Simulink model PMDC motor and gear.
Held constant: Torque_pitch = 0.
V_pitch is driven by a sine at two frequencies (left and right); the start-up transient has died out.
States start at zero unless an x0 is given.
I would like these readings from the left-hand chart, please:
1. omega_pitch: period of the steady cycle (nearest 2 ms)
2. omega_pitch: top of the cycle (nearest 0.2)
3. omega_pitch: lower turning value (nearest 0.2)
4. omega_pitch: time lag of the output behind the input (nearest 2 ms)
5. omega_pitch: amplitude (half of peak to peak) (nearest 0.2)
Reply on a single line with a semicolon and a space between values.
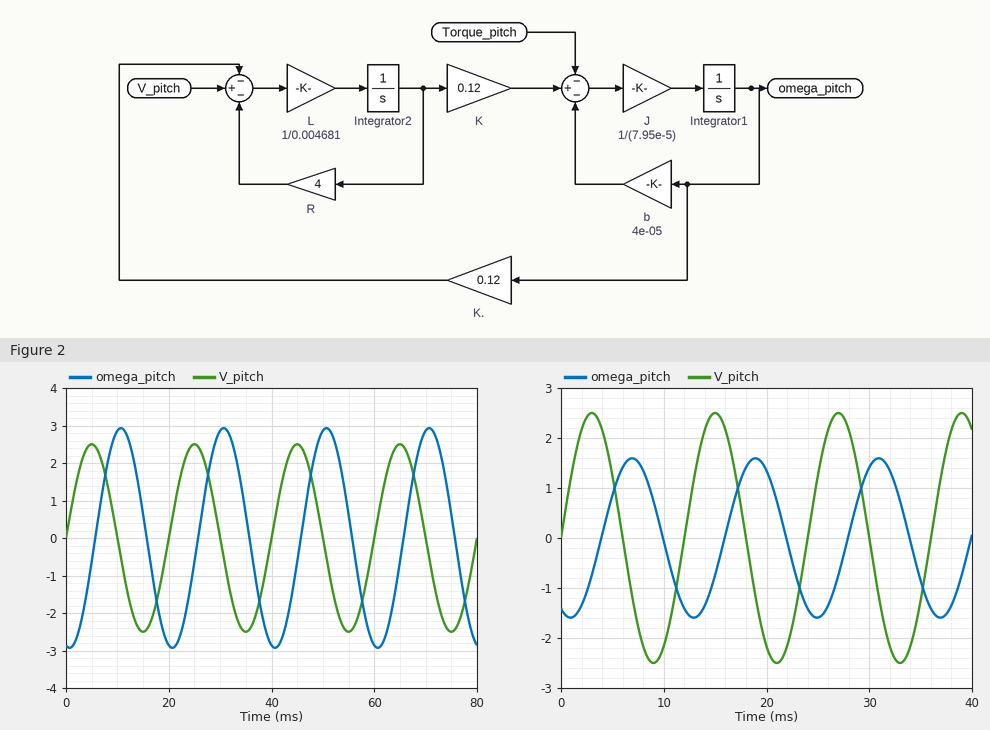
20 ms; 3.0; -3.0; 6 ms; 3.0
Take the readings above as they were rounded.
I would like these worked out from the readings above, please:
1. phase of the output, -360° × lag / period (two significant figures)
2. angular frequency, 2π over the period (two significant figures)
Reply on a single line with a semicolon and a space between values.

-110°; 0.31 rad/ms
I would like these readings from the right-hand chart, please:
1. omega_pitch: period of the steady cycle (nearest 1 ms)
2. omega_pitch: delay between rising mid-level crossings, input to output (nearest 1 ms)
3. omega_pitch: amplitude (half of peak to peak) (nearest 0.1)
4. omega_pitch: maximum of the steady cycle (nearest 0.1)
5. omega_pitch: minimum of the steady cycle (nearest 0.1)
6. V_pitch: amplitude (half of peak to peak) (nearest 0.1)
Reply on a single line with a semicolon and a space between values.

12 ms; 4 ms; 1.6; 1.6; -1.6; 2.5
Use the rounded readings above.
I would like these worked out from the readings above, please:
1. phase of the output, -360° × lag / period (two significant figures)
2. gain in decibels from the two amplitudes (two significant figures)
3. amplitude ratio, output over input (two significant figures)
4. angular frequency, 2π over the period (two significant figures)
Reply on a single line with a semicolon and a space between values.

-120°; -3.9 dB; 0.64; 0.52 rad/ms
